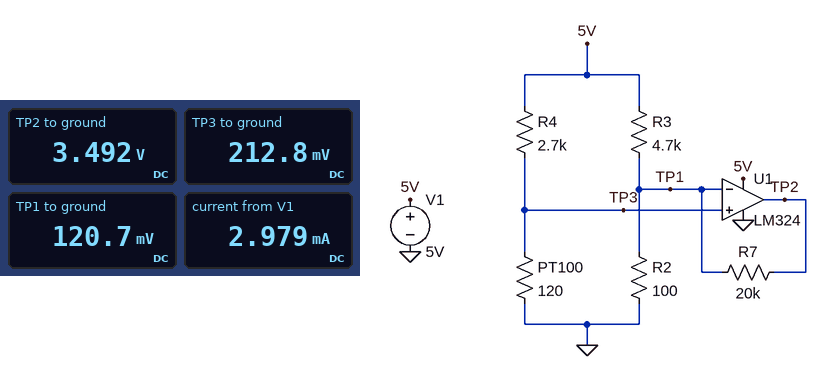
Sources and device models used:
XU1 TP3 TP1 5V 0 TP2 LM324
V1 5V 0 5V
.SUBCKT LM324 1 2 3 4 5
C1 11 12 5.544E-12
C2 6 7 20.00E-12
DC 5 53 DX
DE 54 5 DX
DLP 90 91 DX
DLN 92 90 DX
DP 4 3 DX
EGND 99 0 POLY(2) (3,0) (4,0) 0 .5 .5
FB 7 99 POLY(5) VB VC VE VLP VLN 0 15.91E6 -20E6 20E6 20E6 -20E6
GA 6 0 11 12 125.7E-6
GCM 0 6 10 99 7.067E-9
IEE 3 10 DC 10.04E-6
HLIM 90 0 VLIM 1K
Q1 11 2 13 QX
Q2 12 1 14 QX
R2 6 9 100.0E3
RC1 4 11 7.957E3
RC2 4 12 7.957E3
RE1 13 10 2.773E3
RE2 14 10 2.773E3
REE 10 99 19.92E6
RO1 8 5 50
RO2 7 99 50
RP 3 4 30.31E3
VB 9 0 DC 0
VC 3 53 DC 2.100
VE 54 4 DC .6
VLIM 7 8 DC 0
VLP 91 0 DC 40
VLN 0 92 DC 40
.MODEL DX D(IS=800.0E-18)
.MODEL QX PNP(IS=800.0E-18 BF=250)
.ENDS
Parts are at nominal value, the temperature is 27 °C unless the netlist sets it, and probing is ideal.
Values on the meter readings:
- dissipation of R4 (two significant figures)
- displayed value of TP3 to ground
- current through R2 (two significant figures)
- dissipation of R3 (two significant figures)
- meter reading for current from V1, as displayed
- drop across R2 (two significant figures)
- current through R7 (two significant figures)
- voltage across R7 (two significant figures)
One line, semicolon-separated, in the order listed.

8.5 mW; 212.8 mV; 1.2 mA; 5.1 mW; 2.979 mA; 120 mV; 170 µA; 3.4 V
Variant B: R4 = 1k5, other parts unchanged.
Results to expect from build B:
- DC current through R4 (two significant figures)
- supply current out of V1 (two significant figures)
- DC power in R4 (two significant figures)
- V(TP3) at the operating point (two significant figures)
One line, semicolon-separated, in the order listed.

3.1 mA; 4.3 mA; 14 mW; 370 mV
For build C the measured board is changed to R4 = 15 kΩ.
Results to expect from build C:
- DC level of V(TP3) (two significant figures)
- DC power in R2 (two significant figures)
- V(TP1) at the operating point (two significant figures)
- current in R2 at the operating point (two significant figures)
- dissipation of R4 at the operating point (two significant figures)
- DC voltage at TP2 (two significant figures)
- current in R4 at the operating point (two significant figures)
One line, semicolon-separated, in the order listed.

40 mV; 110 µW; 100 mV; 1.0 mA; 1.6 mW; 14 mV; 330 µA
